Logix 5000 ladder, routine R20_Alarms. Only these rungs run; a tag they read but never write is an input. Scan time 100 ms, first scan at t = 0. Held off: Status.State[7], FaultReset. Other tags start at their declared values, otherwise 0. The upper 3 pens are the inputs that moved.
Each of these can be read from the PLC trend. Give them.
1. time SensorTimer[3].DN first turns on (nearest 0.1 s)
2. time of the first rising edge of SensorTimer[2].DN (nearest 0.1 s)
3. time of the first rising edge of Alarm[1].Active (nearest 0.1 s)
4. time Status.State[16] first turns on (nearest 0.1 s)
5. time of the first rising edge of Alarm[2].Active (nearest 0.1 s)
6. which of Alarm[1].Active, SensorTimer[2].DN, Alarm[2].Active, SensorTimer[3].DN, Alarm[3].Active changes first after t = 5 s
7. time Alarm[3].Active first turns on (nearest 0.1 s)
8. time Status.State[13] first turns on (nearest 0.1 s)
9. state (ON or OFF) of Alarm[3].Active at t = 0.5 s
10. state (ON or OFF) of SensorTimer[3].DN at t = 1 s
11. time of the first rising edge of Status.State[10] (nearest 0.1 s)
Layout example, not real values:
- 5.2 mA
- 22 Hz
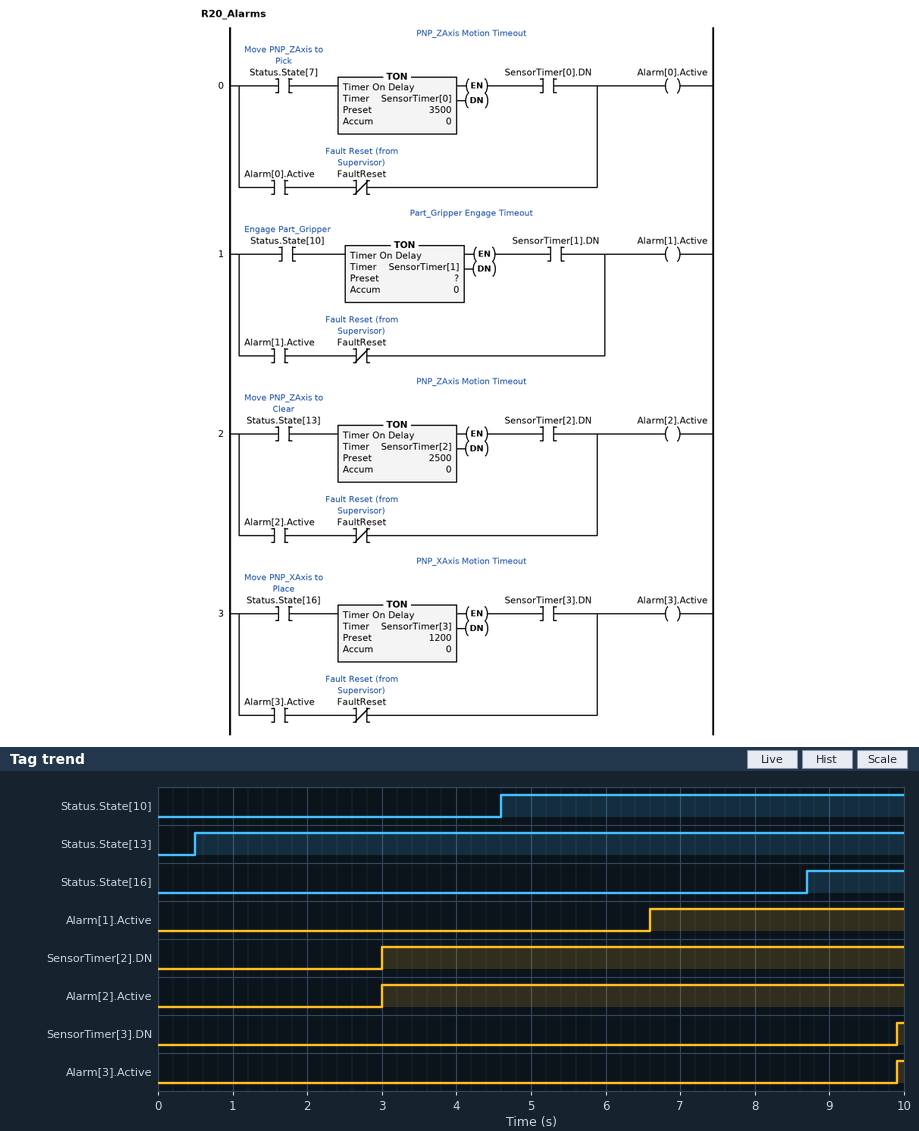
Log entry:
- 9.9 s
- 3.0 s
- 6.6 s
- 8.7 s
- 3.0 s
- Alarm[1].Active
- 9.9 s
- 0.5 s
- OFF
- OFF
- 4.6 s
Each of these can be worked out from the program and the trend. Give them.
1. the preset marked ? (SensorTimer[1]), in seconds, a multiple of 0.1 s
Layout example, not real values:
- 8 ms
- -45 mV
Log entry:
- 2.0 s
